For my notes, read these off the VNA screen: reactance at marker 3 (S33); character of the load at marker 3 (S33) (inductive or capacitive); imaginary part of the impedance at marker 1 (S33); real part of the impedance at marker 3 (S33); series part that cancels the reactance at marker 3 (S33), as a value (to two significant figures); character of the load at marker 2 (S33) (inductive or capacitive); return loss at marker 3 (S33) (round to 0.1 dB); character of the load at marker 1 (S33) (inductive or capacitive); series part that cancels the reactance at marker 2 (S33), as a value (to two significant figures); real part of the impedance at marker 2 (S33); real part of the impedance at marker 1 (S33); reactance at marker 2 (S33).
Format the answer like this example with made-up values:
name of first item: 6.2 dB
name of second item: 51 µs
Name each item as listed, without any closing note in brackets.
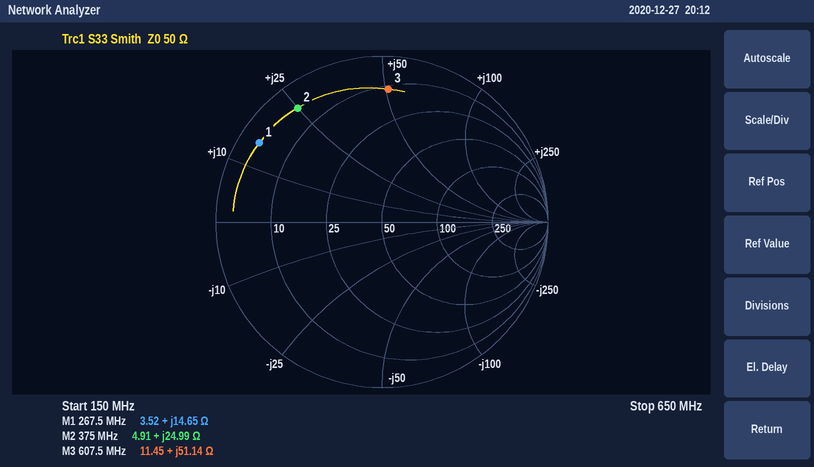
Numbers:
reactance at marker 3: +51.14 Ω
character of the load at marker 3 (S33): inductive
imaginary part of the impedance at marker 1: +14.65 Ω
real part of the impedance at marker 3: 11.45 Ω
series part that cancels the reactance at marker 3 (S33), as a value: 5.1 pF
character of the load at marker 2 (S33): inductive
return loss at marker 3 (S33): 1.9 dB
character of the load at marker 1 (S33): inductive
series part that cancels the reactance at marker 2 (S33), as a value: 17 pF
real part of the impedance at marker 2: 4.91 Ω
real part of the impedance at marker 1: 3.52 Ω
reactance at marker 2: +24.99 Ω
